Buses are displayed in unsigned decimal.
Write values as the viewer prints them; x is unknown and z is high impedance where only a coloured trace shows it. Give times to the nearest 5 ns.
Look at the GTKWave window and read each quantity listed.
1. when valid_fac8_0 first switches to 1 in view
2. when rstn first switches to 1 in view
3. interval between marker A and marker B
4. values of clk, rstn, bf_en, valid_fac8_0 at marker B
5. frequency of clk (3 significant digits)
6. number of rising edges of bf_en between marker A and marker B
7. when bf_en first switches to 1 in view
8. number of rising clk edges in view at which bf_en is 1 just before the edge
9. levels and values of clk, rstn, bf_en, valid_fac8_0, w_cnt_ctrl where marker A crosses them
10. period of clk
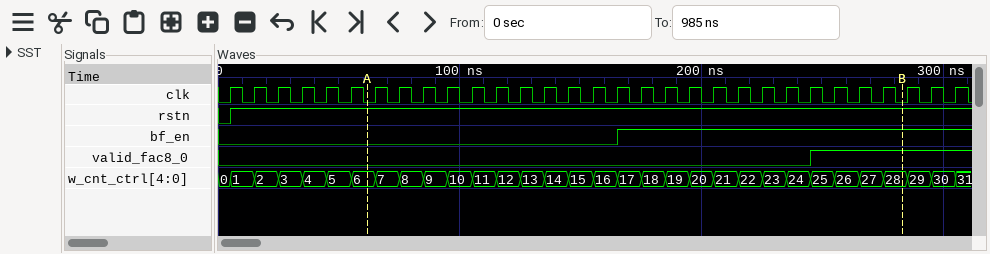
245 ns
5 ns
220 ns
clk=0, rstn=1, bf_en=1, valid_fac8_0=1
100 MHz
1
165 ns
14
clk=0, rstn=1, bf_en=0, valid_fac8_0=0, w_cnt_ctrl=6
10 ns
